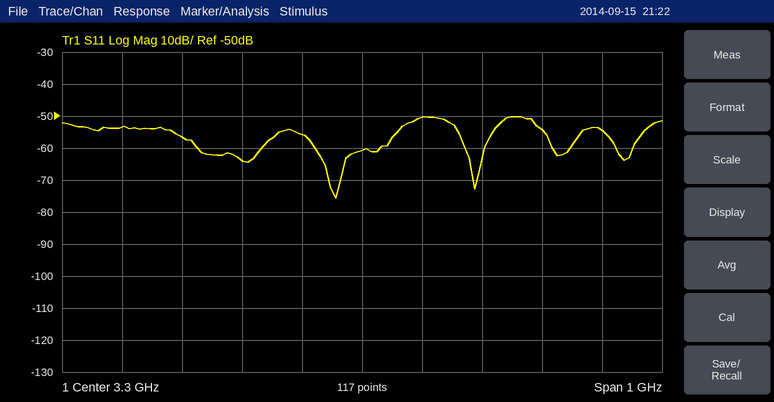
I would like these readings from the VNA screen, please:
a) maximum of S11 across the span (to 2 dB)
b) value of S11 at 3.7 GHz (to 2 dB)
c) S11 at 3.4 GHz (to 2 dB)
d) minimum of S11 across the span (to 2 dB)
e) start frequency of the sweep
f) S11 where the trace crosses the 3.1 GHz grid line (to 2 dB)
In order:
-50 dB
-54 dB
-50 dB
-76 dB
2.8 GHz
-64 dB
